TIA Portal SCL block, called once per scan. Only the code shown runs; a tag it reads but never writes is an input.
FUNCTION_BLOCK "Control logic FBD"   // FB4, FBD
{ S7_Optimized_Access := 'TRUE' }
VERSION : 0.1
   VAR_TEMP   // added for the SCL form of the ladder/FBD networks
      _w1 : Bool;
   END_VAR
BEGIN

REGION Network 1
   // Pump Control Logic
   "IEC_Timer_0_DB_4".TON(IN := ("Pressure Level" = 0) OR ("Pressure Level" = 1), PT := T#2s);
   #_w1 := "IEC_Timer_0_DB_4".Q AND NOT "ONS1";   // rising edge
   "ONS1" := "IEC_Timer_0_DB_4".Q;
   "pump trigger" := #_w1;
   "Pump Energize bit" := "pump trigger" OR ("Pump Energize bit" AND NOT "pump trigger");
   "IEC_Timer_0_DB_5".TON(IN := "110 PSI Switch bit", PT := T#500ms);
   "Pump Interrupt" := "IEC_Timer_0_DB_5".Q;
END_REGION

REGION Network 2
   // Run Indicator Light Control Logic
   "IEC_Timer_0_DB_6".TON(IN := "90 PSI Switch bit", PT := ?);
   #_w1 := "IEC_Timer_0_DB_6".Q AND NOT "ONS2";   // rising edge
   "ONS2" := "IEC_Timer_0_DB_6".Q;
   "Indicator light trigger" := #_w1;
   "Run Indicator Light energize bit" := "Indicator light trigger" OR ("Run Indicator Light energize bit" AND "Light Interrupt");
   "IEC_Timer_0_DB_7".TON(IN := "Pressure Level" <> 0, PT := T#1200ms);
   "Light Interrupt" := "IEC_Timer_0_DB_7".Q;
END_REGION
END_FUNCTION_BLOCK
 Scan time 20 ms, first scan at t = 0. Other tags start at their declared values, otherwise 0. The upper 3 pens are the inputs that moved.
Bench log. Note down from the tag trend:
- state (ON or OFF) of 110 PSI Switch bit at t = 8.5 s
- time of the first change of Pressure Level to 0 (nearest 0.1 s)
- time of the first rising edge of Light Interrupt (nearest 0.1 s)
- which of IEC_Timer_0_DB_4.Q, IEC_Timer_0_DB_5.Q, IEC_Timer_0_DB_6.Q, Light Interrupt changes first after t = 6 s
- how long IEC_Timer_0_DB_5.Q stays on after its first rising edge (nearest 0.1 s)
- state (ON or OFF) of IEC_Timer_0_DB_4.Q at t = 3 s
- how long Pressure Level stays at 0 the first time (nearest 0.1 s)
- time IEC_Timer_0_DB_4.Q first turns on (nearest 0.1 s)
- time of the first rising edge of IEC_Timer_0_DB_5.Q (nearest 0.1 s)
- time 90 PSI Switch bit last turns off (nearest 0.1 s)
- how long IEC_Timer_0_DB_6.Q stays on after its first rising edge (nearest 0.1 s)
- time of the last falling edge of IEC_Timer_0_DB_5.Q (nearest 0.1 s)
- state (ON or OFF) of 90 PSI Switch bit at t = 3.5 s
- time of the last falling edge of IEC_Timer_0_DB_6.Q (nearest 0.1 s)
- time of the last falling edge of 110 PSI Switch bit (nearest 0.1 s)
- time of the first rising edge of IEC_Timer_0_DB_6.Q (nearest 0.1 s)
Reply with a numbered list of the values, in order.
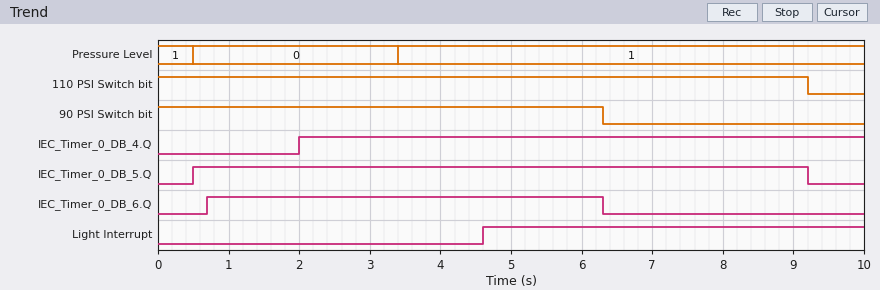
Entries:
1. ON
2. 0.5 s
3. 4.6 s
4. IEC_Timer_0_DB_6.Q
5. 8.7 s
6. ON
7. 2.9 s
8. 2.0 s
9. 0.5 s
10. 6.3 s
11. 5.6 s
12. 9.2 s
13. ON
14. 6.3 s
15. 9.2 s
16. 0.7 s
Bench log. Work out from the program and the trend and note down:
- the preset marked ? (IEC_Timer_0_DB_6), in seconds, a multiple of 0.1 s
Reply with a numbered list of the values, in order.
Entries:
1. 0.7 s
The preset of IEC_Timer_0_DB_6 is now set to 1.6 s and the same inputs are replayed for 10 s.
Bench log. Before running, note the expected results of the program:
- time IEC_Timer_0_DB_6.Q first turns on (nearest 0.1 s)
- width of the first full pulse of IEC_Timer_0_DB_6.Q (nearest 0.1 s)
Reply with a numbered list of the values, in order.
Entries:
1. 1.6 s
2. 4.7 s
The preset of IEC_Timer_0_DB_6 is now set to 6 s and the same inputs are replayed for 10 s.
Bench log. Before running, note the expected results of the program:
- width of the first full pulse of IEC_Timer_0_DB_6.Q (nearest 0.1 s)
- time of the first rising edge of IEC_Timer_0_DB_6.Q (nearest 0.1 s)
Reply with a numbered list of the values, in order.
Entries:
1. 0.3 s
2. 6.0 s
